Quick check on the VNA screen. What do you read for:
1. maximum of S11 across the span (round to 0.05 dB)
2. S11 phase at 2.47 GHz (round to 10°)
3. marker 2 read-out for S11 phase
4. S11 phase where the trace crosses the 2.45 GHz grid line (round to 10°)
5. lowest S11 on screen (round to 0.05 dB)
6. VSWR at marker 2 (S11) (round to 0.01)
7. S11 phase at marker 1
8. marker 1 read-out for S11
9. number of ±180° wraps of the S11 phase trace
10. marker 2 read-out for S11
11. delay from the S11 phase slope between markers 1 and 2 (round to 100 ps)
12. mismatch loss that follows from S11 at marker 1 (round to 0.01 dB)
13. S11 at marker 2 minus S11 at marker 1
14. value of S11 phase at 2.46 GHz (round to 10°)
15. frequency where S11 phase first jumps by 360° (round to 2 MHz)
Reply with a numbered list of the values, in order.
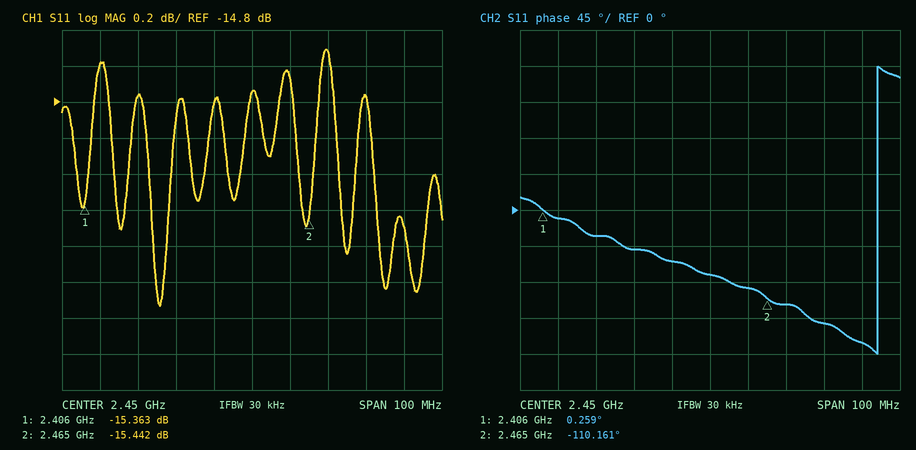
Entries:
1. -14.50 dB
2. -120°
3. -110.161°
4. -80°
5. -15.95 dB
6. 1.41
7. 0.259°
8. -15.363 dB
9. 1
10. -15.442 dB
11. 5.2 ns
12. 0.13 dB
13. -0.079 dB
14. -100°
15. 2.494 GHz
